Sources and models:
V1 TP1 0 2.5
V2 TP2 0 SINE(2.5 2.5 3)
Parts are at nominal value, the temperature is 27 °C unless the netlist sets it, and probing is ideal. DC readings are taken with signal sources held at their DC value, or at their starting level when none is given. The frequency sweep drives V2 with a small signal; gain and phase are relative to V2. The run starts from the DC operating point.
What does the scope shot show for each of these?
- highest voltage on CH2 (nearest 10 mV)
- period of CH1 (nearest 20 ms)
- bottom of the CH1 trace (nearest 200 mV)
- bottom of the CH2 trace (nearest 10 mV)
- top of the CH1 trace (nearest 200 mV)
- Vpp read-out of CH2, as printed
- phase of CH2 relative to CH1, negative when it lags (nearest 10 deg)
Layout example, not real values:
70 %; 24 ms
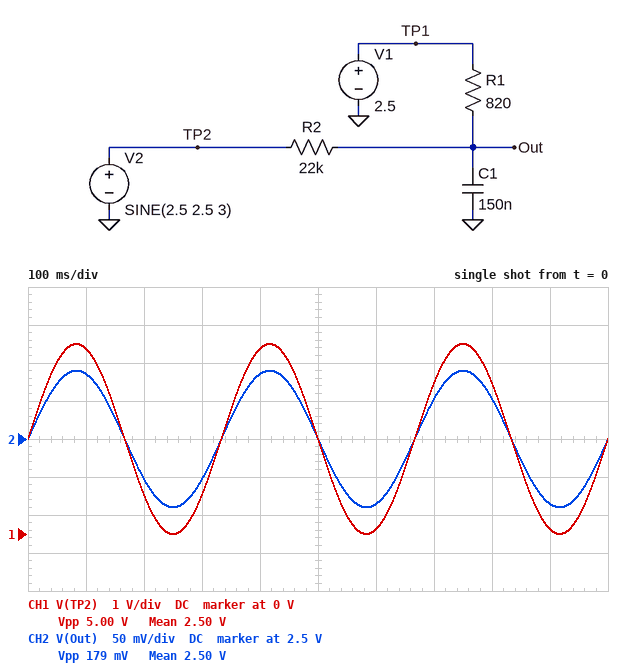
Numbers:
2.59 V; 340 ms; 0 V; 2.41 V; 5.0 V; 179 mV; 0 deg
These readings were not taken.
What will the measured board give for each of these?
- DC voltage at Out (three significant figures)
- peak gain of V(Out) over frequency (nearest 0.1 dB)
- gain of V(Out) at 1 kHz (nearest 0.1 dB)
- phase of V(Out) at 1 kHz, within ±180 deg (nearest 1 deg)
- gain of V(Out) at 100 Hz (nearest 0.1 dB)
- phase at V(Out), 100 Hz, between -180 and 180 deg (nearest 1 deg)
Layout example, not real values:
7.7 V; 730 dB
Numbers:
2.50 V; -28.9 dB; -30.8 dB; -37 deg; -28.9 dB; -4 deg
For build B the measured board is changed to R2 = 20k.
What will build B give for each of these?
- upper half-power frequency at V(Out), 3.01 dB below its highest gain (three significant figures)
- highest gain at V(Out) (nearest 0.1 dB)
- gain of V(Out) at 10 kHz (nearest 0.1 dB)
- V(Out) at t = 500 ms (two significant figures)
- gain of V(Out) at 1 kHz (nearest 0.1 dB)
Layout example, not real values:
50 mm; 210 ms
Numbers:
1.35 kHz; -28.1 dB; -45.6 dB; 2.5 V; -30.0 dB
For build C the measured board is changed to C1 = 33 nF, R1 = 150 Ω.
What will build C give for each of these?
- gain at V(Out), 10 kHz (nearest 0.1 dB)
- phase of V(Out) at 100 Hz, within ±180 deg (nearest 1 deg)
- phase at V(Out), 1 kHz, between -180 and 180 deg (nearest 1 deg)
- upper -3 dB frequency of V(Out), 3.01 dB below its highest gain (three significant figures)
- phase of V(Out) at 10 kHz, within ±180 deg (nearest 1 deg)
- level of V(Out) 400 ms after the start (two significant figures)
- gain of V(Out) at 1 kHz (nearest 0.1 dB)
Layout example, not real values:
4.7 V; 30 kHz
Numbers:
-43.8 dB; 0 deg; -2 deg; 32.4 kHz; -17 deg; 2.5 V; -43.4 dB
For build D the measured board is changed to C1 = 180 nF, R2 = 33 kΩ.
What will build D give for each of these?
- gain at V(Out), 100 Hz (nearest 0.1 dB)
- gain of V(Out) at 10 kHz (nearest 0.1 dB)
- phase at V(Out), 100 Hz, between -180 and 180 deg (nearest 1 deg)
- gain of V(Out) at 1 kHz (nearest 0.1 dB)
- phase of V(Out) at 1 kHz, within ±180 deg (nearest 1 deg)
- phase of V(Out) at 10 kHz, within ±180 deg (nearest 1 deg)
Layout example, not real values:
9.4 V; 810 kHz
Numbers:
-32.3 dB; -51.5 dB; -5 deg; -34.9 dB; -42 deg; -84 deg
